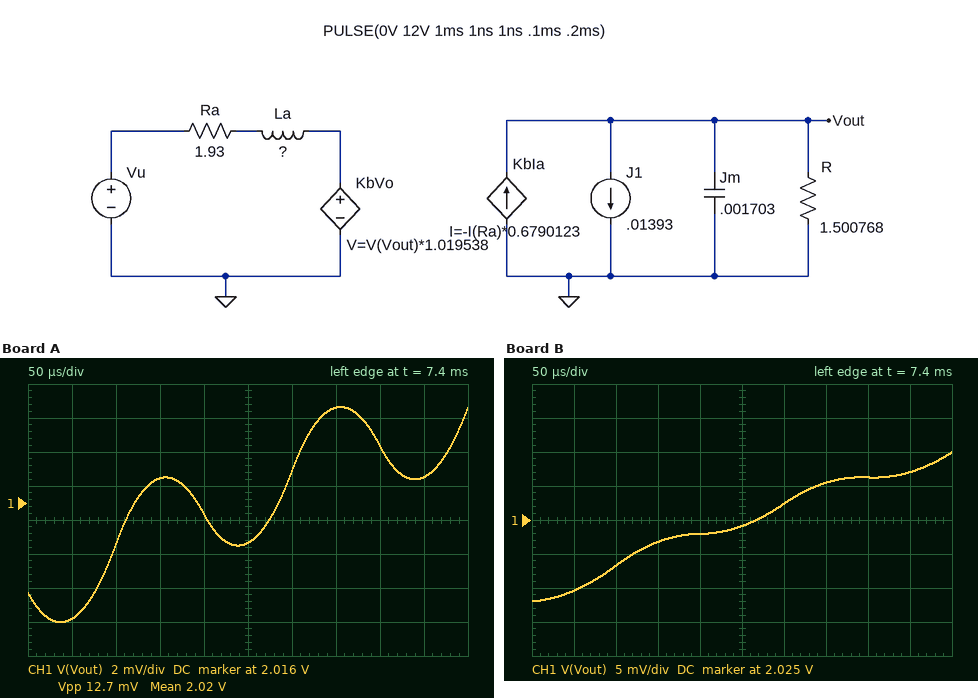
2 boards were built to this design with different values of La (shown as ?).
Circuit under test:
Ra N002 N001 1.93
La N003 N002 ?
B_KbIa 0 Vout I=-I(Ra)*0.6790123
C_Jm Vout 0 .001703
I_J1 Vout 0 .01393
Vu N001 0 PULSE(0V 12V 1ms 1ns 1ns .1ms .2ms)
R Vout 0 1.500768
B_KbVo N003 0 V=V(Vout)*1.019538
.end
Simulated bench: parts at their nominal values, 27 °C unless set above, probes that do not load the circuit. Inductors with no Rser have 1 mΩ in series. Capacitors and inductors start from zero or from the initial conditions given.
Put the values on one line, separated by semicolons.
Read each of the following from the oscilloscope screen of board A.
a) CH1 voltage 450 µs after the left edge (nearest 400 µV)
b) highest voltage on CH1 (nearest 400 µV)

2.0176 V; 2.0216 V
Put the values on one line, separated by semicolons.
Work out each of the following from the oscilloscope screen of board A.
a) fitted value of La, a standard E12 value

1 mH
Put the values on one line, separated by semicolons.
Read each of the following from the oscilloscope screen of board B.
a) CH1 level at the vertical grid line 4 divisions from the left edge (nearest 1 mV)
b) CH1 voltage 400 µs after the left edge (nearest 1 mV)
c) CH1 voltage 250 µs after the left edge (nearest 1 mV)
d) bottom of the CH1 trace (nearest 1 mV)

2.023 V; 2.031 V; 2.024 V; 2.013 V
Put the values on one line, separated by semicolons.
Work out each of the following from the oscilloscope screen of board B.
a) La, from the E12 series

2.7 mH
